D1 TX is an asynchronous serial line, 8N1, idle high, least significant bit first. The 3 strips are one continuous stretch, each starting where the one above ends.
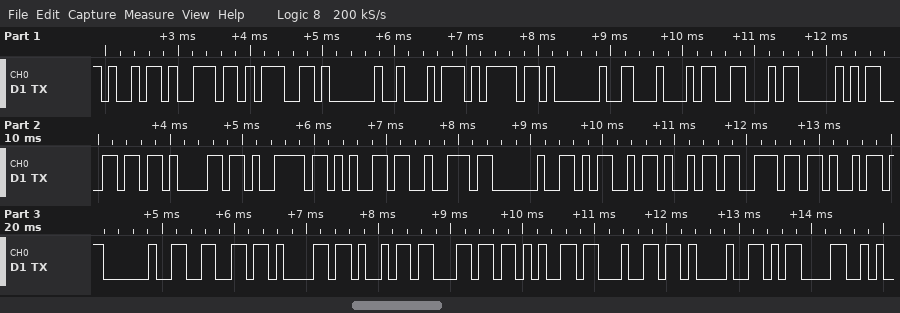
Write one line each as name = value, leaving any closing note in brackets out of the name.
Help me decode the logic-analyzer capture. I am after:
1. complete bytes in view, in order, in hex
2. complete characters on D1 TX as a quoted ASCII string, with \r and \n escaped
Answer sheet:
complete bytes in view, in order, in hex = 69 6E 67 20 74 6F 20 44 46 50 6C 61 79 65 72 20 4D 69 6E 69 20 66 61 69 6C 65 64 21 0D
complete characters on D1 TX as a quoted ASCII string, with \r and \n escaped = "ing to DFPlayer Mini failed!\r"
